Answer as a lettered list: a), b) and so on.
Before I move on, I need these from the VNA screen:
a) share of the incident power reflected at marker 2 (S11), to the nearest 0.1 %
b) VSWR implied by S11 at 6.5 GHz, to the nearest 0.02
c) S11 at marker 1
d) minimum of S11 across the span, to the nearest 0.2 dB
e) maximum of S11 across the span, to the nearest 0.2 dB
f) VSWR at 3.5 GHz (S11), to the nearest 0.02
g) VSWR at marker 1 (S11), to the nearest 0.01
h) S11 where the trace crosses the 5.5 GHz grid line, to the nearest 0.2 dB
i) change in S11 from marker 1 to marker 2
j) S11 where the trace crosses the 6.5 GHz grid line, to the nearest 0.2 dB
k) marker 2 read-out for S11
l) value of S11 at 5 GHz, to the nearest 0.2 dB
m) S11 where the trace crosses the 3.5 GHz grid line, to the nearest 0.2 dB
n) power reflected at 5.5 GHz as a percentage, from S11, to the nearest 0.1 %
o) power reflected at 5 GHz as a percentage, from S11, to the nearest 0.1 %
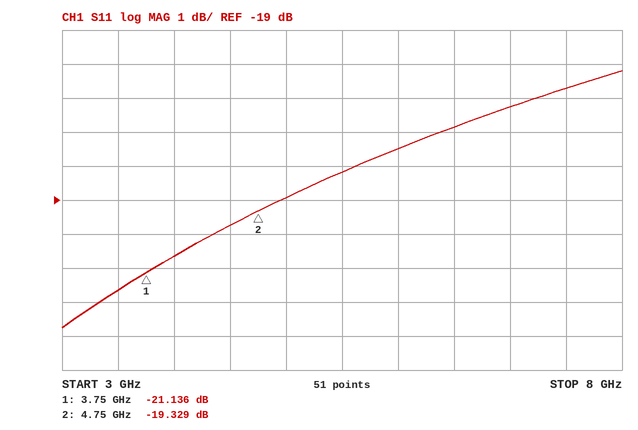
a) 1.2 %
b) 1.34
c) -21.136 dB
d) -22.8 dB
e) -15.2 dB
f) 1.18
g) 1.19
h) -18.2 dB
i) 1.807 dB
j) -16.8 dB
k) -19.329 dB
l) -19.0 dB
m) -21.6 dB
n) 1.5 %
o) 1.3 %
